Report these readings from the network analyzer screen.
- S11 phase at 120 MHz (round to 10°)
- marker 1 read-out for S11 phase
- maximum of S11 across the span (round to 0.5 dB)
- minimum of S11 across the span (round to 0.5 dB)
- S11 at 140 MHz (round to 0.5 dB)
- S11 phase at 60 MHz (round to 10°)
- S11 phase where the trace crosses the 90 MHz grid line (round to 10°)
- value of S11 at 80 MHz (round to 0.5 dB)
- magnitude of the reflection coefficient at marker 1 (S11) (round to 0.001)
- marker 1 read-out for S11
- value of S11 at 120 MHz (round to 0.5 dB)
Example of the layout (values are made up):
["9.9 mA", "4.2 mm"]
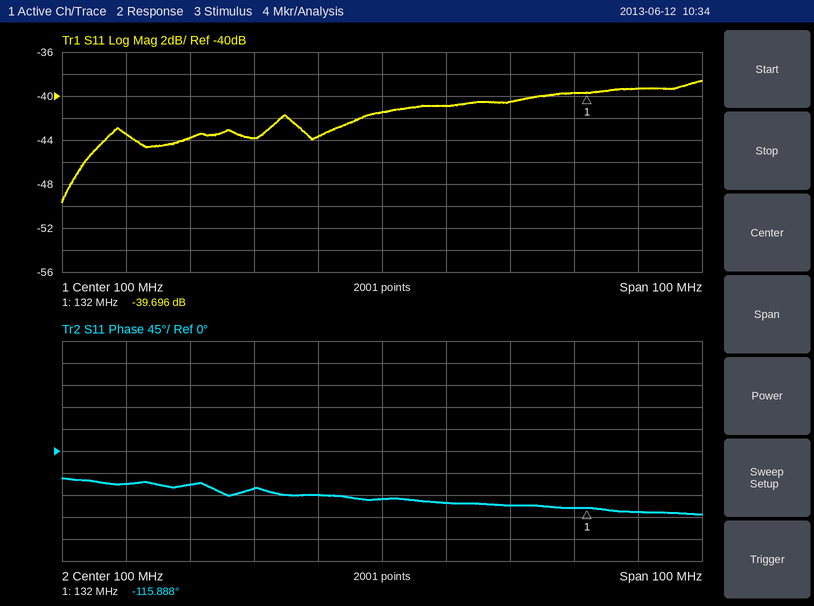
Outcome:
["-110°", "-115.888°", "-38.5 dB", "-49.5 dB", "-39.5 dB", "-70°", "-90°", "-44.0 dB", "0.010", "-39.696 dB", "-40.5 dB"]
